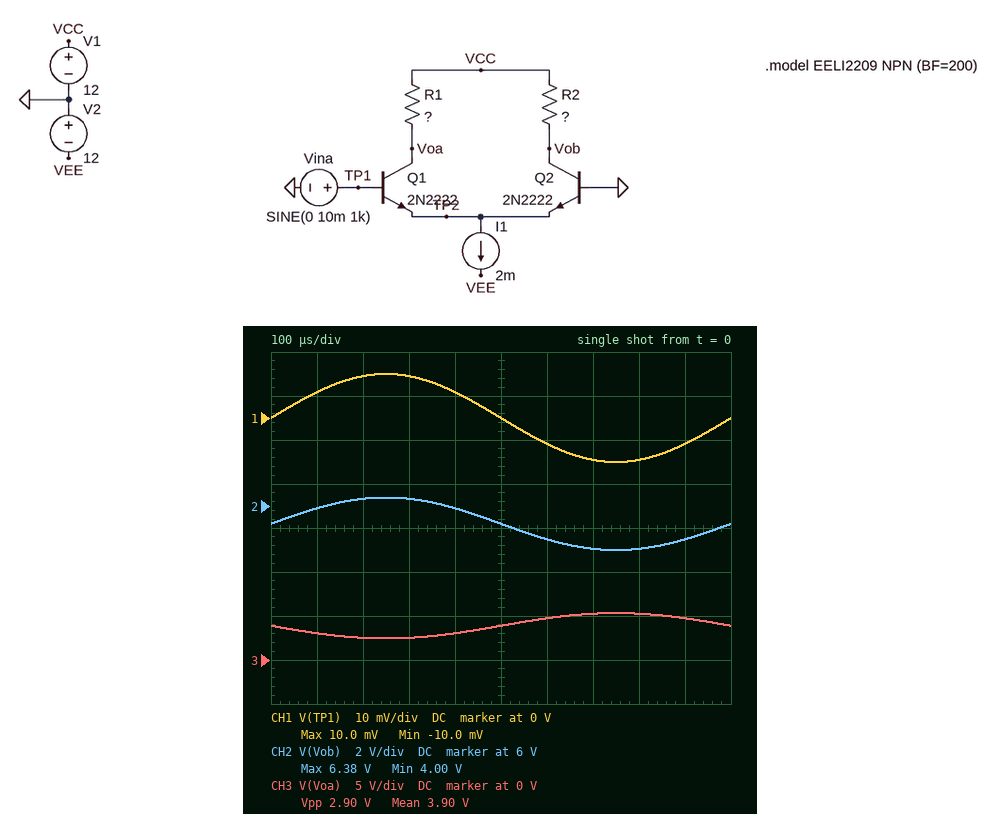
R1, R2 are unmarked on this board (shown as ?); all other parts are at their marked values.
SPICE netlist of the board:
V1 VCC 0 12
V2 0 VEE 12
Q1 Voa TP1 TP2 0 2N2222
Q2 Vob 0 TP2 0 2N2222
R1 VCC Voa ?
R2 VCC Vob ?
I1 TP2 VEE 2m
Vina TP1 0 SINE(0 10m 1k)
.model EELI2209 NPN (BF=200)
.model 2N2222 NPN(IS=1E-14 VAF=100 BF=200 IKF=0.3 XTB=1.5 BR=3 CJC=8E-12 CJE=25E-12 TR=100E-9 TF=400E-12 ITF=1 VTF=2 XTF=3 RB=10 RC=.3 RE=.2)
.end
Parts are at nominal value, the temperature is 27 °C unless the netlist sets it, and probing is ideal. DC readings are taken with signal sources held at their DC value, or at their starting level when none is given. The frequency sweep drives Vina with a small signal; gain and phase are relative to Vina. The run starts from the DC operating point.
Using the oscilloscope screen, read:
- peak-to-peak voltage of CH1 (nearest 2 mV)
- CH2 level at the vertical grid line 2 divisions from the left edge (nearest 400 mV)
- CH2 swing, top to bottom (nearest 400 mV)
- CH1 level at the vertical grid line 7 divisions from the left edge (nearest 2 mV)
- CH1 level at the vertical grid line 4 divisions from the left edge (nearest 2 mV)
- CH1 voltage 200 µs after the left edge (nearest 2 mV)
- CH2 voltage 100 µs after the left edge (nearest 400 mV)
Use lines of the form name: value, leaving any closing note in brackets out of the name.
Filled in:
peak-to-peak voltage of CH1: 20 mV
CH2 level at the vertical grid line 2 divisions from the left edge: 6.4 V
CH2 swing, top to bottom: 2.4 V
CH1 level at the vertical grid line 7 divisions from the left edge: -10 mV
CH1 level at the vertical grid line 4 divisions from the left edge: 6 mV
CH1 voltage 200 µs after the left edge: 10 mV
CH2 voltage 100 µs after the left edge: 6.0 V
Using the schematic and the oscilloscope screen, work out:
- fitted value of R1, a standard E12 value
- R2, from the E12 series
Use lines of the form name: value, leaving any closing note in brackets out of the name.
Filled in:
fitted value of R1, a standard E12 value: 8.2 kΩ
R2, from the E12 series: 6.8 kΩ
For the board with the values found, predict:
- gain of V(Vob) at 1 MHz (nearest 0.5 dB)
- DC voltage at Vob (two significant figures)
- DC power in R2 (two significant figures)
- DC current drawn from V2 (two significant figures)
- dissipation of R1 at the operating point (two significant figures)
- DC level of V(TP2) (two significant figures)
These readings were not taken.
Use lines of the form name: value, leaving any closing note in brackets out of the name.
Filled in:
gain of V(Vob) at 1 MHz: 41.5 dB
DC voltage at Vob: 5.2 V
DC power in R2: 6.8 mW
DC current drawn from V2: 2.0 mA
dissipation of R1 at the operating point: 8.0 mW
DC level of V(TP2): -650 mV
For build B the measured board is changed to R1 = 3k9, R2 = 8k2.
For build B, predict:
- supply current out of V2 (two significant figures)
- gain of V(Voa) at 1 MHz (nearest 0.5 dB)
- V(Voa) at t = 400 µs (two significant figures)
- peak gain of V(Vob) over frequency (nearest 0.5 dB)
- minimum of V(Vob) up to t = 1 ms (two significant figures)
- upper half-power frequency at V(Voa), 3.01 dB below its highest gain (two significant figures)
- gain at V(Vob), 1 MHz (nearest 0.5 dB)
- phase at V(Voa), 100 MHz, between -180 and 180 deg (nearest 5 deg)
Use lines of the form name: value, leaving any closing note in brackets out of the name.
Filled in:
supply current out of V2: 2.0 mA
gain of V(Voa) at 1 MHz: 37.0 dB
V(Voa) at t = 400 µs: 7.6 V
peak gain of V(Vob) over frequency: 43.5 dB
minimum of V(Vob) up to t = 1 ms: 2.5 V
upper half-power frequency at V(Voa), 3.01 dB below its highest gain: 7.8 MHz
gain at V(Vob), 1 MHz: 43.0 dB
phase at V(Voa), 100 MHz, between -180 and 180 deg: 75 deg
